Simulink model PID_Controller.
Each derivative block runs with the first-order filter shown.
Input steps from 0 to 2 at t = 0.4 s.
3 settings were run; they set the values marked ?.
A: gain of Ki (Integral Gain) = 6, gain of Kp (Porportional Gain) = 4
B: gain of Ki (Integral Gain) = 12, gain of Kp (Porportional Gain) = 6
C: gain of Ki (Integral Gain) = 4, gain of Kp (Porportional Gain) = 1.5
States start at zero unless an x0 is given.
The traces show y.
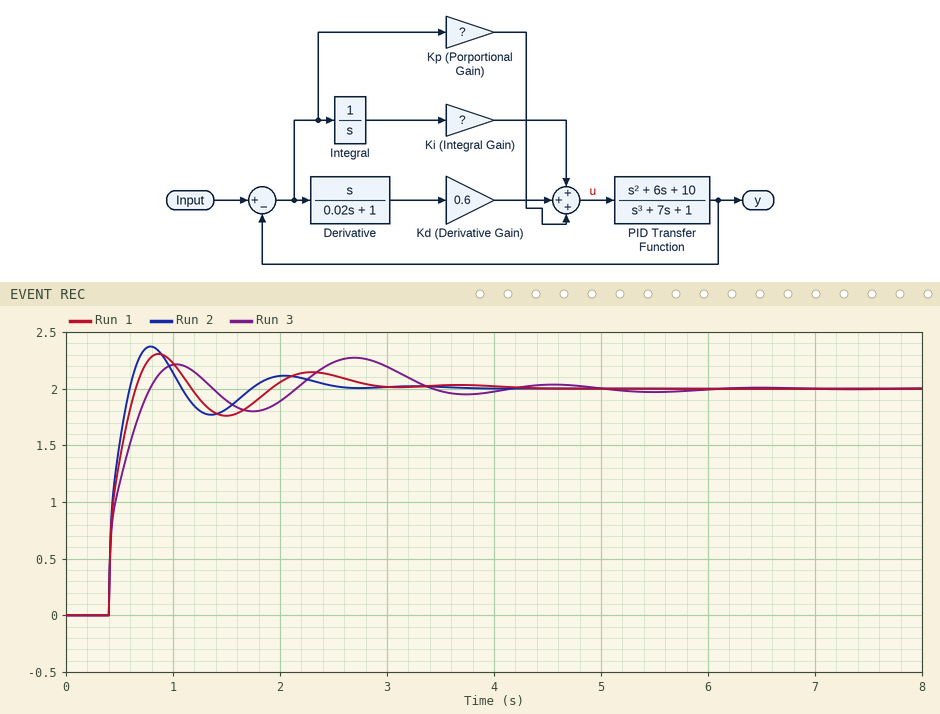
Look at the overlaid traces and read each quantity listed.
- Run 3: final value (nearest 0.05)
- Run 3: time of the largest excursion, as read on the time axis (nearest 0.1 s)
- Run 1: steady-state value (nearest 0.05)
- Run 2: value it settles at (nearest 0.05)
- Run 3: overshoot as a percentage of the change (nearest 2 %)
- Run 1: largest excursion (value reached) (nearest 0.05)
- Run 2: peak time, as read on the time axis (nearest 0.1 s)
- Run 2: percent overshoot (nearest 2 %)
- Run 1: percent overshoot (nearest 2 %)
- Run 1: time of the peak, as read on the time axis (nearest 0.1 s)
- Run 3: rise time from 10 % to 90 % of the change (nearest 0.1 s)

2.00
2.7 s
2.00
2.00
14 %
2.30
0.8 s
18 %
16 %
0.9 s
0.3 s
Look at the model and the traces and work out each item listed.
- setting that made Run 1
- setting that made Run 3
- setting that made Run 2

A
C
B
